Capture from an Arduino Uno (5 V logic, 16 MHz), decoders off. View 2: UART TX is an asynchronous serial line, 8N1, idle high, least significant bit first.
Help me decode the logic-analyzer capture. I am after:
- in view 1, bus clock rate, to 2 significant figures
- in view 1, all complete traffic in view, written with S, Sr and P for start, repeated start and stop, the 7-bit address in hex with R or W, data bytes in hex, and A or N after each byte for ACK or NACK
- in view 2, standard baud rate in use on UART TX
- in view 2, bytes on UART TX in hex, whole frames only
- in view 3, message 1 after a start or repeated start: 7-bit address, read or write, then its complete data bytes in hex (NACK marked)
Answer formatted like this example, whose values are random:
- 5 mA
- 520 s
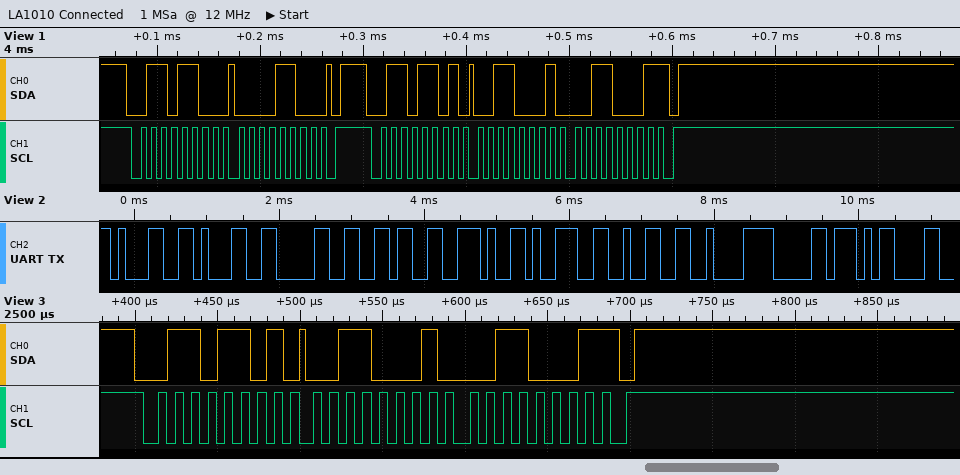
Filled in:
- 100 kHz
- S 36W A 0C A P S 36R A 31 A 31 N P
- 9600 baud
- 31 31 30 36 2E 39 32 C2 B0 0D
- 0x36 read: 31 31 NACK
